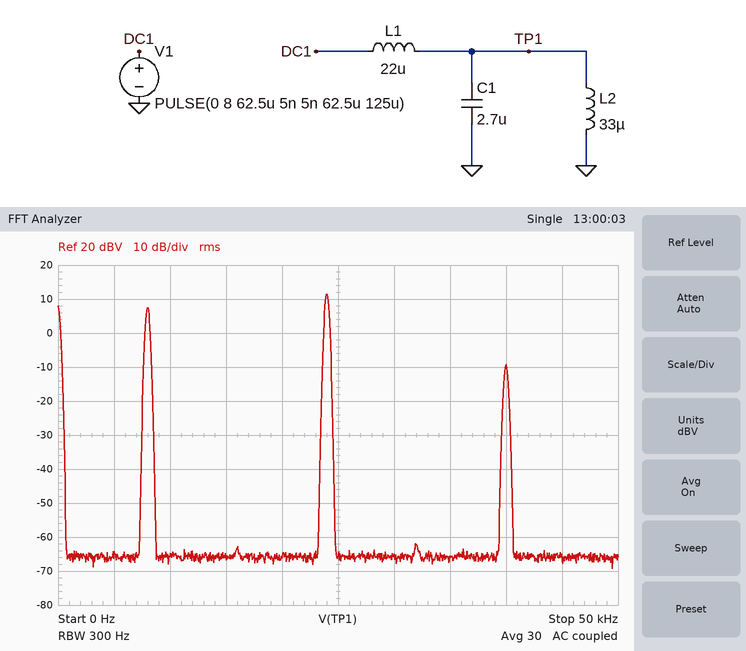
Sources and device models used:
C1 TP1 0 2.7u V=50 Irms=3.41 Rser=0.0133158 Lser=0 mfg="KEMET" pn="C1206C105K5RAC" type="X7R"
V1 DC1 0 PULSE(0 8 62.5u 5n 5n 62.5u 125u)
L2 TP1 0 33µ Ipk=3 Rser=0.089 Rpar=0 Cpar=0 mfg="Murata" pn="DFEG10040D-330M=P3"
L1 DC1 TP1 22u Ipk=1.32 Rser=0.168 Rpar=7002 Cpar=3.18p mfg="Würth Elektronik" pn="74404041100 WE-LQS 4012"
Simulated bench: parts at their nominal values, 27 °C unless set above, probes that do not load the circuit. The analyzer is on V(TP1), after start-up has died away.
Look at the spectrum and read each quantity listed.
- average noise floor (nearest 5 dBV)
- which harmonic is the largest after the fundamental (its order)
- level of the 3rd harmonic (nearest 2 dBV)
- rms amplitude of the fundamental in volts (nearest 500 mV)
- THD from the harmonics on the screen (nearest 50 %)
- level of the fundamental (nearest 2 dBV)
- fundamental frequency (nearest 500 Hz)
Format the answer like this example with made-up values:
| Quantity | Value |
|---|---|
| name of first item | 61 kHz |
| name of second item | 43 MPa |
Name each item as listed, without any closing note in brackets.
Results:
| Quantity | Value |
|---|---|
| average noise floor | -65 dBV |
| which harmonic is the largest after the fundamental | 3 |
| level of the 3rd harmonic | 12 dBV |
| rms amplitude of the fundamental in volts | 2.5 V |
| THD from the harmonics on the screen | 150 % |
| level of the fundamental | 8 dBV |
| fundamental frequency | 8.0 kHz |
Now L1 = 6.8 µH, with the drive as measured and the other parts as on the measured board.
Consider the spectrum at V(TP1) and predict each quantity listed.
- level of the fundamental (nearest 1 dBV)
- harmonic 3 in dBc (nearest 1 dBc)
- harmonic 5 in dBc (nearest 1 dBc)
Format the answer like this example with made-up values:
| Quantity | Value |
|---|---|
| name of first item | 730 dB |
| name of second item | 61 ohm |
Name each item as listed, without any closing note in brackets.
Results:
| Quantity | Value |
|---|---|
| level of the fundamental | 10 dBV |
| harmonic 3 in dBc | -6 dBc |
| harmonic 5 in dBc | 6 dBc |
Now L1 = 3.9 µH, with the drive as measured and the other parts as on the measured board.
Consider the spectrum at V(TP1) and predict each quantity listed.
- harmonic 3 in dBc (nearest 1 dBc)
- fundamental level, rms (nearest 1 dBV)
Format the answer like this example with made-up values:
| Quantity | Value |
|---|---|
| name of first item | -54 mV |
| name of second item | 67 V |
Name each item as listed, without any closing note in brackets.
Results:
| Quantity | Value |
|---|---|
| harmonic 3 in dBc | -8 dBc |
| fundamental level, rms | 10 dBV |
